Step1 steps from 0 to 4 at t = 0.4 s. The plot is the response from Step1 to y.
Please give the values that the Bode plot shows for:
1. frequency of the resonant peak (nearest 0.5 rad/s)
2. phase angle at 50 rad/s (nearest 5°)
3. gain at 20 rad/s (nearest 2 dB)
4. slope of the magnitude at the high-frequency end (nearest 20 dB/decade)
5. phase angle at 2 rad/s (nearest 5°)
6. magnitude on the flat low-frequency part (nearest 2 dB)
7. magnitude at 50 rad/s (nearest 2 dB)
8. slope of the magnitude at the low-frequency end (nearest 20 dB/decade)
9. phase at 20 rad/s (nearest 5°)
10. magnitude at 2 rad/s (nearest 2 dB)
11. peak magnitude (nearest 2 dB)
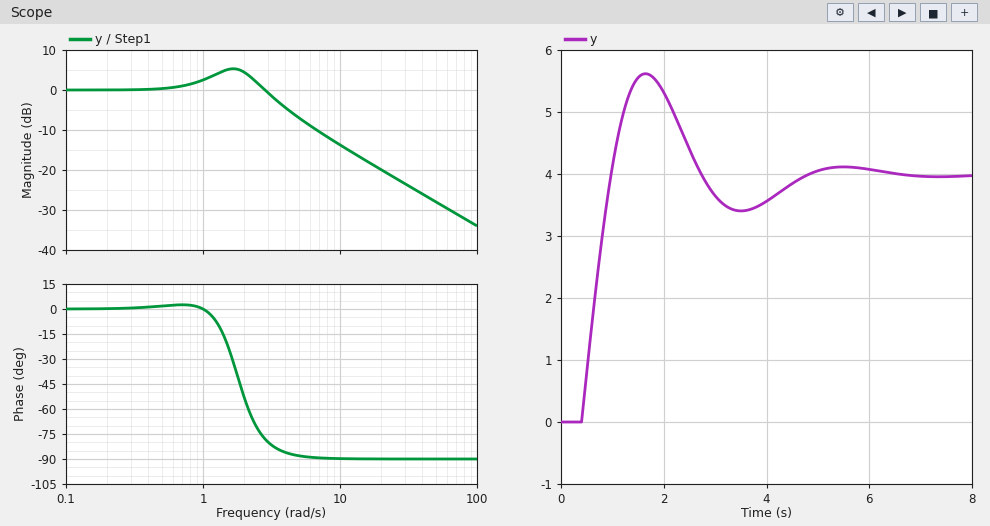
1.5 rad/s
-90°
-20 dB
-20 dB/decade
-55°
0 dB
-28 dB
0 dB/decade
-90°
4 dB
6 dB
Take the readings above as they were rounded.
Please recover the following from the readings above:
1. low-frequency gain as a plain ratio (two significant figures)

1.0
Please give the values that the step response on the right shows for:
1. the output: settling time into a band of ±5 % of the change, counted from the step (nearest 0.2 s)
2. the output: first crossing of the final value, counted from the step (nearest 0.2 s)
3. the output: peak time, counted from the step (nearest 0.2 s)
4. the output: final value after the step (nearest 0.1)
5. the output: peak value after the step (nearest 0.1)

4.0 s
0.6 s
1.2 s
4.0
5.6
